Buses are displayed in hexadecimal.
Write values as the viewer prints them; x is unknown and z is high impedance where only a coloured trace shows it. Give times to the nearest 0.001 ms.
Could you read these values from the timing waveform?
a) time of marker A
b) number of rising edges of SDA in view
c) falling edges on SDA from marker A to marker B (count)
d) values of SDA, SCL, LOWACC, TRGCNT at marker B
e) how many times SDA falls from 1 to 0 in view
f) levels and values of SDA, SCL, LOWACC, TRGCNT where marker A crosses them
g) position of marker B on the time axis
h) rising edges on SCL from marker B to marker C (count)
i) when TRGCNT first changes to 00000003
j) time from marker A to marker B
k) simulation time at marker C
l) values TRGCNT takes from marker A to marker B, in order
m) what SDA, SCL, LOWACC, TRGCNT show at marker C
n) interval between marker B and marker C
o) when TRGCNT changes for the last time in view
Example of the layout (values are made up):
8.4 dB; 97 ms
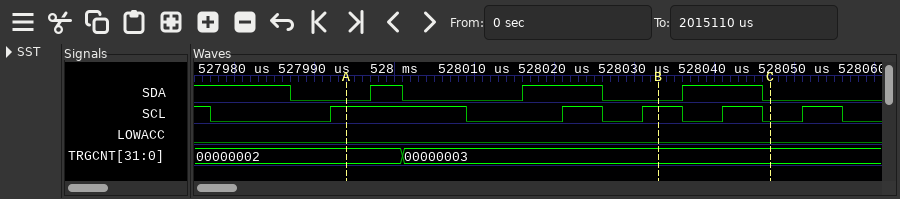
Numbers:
527.994 ms; 3; 2; SDA=0, SCL=1, LOWACC=0, TRGCNT=00000003; 4; SDA=0, SCL=1, LOWACC=0, TRGCNT=00000002; 528.033 ms; 1; 528.001 ms; 0.039 ms; 528.047 ms; 00000002, 00000003; SDA=0, SCL=0, LOWACC=0, TRGCNT=00000003; 0.014 ms; 528.001 ms
